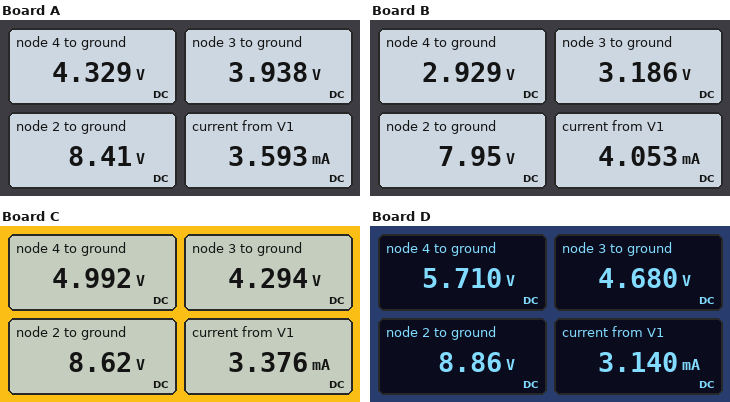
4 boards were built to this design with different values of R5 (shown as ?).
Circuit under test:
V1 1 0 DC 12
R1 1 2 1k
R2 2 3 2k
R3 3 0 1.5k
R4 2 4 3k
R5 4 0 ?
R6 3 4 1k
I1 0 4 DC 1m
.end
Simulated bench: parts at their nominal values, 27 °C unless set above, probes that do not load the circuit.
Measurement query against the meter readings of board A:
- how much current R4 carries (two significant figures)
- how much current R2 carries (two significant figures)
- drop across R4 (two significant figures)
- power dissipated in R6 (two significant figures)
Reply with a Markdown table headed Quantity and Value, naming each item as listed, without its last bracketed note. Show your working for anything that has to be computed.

| Quantity | Value |
|---|---|
| how much current R4 carries | (8.41 V - 4.329 V) / 3 kΩ = 1.4 mA |
| how much current R2 carries | (8.41 V - 3.938 V) / 2 kΩ = 2.2 mA |
| drop across R4 | 8.41 V - 4.329 V = 4.1 V |
| power dissipated in R6 | (4.329 V - 3.938 V)^2 / 1 kΩ = 150 µW |
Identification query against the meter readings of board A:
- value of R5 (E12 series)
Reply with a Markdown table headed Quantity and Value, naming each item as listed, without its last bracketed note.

| Quantity | Value |
|---|---|
| value of R5 | 2.2 kΩ |
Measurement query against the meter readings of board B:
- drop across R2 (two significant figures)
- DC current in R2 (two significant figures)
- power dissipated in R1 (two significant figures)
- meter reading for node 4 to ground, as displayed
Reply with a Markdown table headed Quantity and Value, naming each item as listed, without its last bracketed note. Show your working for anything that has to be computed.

| Quantity | Value |
|---|---|
| drop across R2 | 7.95 V - 3.186 V = 4.8 V |
| DC current in R2 | (7.95 V - 3.186 V) / 2 kΩ = 2.4 mA |
| power dissipated in R1 | (12 V - 7.95 V)^2 / 1 kΩ = 16 mW |
| meter reading for node 4 to ground, as displayed | 2.929 V |
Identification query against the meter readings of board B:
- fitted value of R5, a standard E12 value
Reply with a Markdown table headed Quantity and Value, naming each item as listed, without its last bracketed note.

| Quantity | Value |
|---|---|
| fitted value of R5, a standard E12 value | 1 kΩ |
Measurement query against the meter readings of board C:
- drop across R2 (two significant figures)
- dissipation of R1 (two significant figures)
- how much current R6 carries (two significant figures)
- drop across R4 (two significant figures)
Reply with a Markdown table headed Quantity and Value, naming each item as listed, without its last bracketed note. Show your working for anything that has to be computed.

| Quantity | Value |
|---|---|
| drop across R2 | 8.62 V - 4.294 V = 4.3 V |
| dissipation of R1 | (12 V - 8.62 V)^2 / 1 kΩ = 11 mW |
| how much current R6 carries | (4.992 V - 4.294 V) / 1 kΩ = 700 µA |
| drop across R4 | 8.62 V - 4.992 V = 3.6 V |
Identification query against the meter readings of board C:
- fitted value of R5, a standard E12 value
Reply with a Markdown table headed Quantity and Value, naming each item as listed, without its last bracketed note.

| Quantity | Value |
|---|---|
| fitted value of R5, a standard E12 value | 3.3 kΩ |
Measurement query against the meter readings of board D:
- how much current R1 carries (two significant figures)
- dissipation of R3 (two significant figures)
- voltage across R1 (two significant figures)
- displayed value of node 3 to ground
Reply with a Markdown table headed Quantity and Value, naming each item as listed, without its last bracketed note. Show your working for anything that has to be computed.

| Quantity | Value |
|---|---|
| how much current R1 carries | (12 V - 8.86 V) / 1 kΩ = 3.1 mA |
| dissipation of R3 | (4.68 V)^2 / 1.5 kΩ = 15 mW |
| voltage across R1 | 12 V - 8.86 V = 3.1 V |
| displayed value of node 3 to ground | 4.680 V |
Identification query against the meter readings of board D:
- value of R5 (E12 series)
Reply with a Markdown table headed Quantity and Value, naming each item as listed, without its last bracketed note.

| Quantity | Value |
|---|---|
| value of R5 | 5.6 kΩ |
